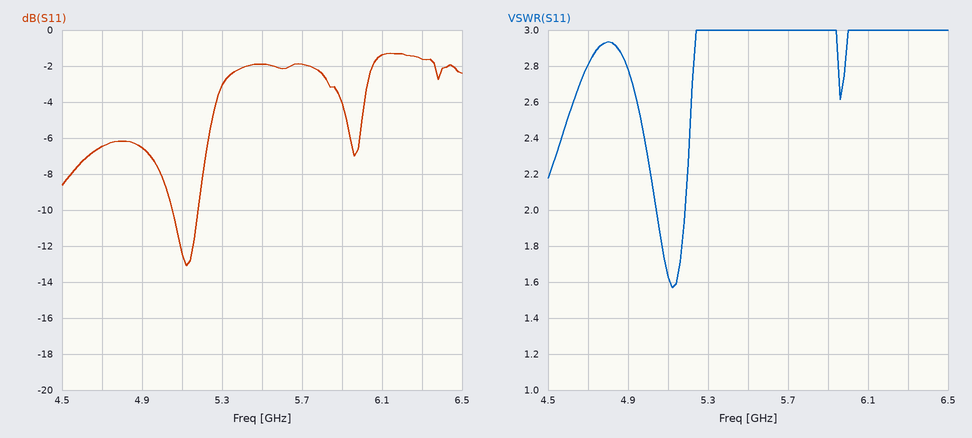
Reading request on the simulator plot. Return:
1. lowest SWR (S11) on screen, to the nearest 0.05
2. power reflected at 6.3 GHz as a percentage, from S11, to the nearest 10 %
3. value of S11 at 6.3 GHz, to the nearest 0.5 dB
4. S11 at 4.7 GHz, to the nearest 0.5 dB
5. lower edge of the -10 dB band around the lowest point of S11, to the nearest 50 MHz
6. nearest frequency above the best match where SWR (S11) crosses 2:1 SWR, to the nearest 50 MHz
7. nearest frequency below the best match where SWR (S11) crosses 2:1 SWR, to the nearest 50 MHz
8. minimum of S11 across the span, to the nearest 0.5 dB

1.55
70 %
-1.5 dB
-6.5 dB
5.05 GHz
5.20 GHz
5.05 GHz
-13.0 dB
